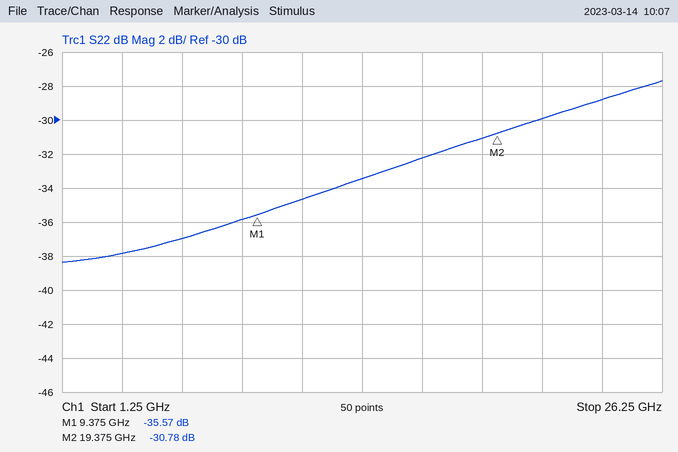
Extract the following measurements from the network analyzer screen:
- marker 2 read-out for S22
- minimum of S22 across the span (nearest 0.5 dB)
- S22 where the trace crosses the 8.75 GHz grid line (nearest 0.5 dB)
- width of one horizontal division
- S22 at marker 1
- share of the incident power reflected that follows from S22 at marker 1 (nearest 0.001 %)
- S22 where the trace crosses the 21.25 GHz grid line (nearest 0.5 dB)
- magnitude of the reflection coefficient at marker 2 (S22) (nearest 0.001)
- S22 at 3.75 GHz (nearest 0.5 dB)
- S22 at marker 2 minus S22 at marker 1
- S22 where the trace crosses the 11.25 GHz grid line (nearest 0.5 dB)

-30.78 dB
-38.5 dB
-36.0 dB
2.5 GHz
-35.57 dB
0.028 %
-30.0 dB
0.029
-38.0 dB
4.79 dB
-34.5 dB
